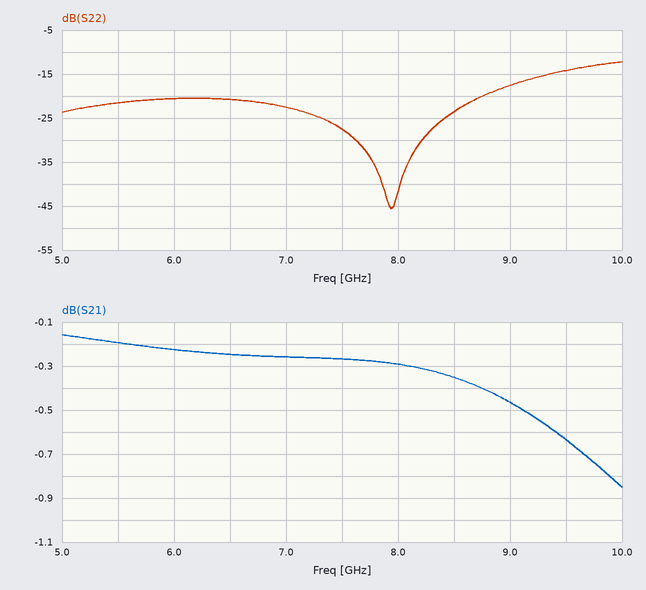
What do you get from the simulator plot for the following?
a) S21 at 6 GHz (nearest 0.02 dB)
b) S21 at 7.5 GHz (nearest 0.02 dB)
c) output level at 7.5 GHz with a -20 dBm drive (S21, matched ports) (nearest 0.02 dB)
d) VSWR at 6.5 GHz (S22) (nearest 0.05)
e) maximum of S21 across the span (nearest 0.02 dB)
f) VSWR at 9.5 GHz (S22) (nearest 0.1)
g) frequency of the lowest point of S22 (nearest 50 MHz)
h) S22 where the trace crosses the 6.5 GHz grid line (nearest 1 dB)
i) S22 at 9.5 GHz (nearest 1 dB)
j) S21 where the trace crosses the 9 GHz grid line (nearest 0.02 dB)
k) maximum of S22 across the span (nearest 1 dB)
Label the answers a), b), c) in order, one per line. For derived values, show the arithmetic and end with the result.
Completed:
a) -0.22 dB
b) -0.26 dB
c) -20 dBm + (-0.26 dB) = -20.26 dBm
d) |Γ| = 10^(-21/20) = 0.0891; VSWR = (1 + 0.0891)/(1 − 0.0891) ≈ 1.20
e) -0.16 dB
f) |Γ| = 10^(-14/20) = 0.1995; VSWR = (1 + 0.1995)/(1 − 0.1995) ≈ 1.5
g) 7.95 GHz
h) -21 dB
i) -14 dB
j) -0.46 dB
k) -12 dB
